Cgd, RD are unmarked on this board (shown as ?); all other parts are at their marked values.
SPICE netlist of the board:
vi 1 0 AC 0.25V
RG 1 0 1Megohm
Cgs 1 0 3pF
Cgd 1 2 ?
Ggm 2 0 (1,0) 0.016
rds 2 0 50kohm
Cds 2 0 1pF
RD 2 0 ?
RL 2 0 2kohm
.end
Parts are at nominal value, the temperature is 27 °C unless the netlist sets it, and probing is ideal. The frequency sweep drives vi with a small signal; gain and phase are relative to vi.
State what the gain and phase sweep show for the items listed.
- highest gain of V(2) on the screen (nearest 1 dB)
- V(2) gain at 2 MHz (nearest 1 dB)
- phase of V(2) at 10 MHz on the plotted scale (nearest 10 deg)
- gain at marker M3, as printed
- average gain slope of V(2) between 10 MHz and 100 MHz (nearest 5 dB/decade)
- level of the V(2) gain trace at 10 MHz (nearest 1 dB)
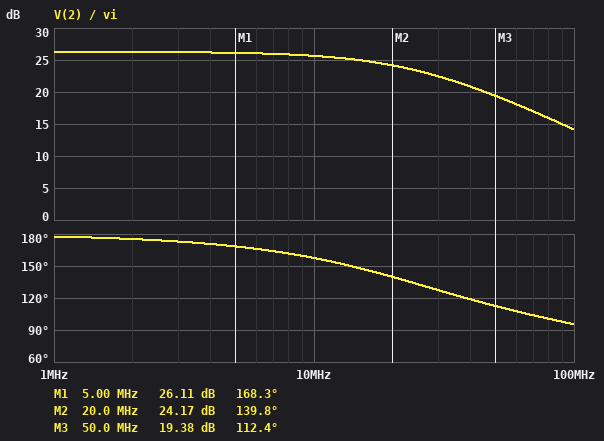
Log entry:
26 dB
26 dB
160 deg
19.38 dB
-10 dB/decade
26 dB
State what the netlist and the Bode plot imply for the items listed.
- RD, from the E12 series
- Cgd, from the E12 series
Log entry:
3.9 kΩ
3.9 pF
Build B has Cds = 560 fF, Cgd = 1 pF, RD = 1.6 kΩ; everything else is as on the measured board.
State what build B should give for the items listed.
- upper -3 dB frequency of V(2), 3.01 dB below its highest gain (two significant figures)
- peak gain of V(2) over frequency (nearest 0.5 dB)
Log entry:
120 MHz
23.0 dB
